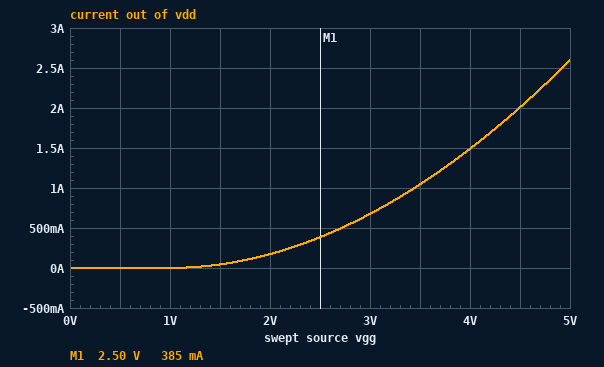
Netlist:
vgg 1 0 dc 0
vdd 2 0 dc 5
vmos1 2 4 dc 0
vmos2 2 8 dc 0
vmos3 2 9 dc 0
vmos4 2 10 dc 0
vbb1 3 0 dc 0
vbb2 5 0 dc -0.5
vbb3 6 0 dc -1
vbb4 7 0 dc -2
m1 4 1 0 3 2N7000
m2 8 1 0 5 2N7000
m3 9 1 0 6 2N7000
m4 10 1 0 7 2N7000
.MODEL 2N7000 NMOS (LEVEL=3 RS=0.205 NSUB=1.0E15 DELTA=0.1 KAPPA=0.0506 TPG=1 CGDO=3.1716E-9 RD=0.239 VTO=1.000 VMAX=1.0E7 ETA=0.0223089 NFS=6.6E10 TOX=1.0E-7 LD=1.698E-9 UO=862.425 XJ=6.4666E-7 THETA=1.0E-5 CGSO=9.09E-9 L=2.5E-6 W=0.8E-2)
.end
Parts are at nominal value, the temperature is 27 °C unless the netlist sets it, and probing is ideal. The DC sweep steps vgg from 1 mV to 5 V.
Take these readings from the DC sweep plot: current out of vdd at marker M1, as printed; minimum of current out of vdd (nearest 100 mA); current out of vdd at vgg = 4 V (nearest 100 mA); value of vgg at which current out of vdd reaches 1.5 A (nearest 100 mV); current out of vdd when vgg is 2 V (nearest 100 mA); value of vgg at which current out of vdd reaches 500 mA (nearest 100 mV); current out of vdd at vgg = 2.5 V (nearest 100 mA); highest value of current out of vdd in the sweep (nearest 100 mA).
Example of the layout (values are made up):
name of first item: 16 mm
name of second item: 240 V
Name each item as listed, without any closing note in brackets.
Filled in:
current out of vdd at marker M1, as printed: 385 mA
minimum of current out of vdd: 0 A
current out of vdd at vgg = 4 V: 1.5 A
value of vgg at which current out of vdd reaches 1.5 A: 4.0 V
current out of vdd when vgg is 2 V: 200 mA
value of vgg at which current out of vdd reaches 500 mA: 2.7 V
current out of vdd at vgg = 2.5 V: 400 mA
highest value of current out of vdd in the sweep: 2.6 A
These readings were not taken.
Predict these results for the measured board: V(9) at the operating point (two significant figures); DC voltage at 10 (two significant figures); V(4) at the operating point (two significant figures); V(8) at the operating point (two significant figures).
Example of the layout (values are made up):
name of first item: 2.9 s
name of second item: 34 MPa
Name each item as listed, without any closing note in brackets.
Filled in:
V(9) at the operating point: 5.0 V
DC voltage at 10: 5.0 V
V(4) at the operating point: 5.0 V
V(8) at the operating point: 5.0 V
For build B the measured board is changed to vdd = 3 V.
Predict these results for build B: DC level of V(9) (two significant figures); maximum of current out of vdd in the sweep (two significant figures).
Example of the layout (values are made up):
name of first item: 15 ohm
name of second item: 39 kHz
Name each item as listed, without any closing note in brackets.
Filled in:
DC level of V(9): 3.0 V
maximum of current out of vdd in the sweep: 2.5 A
